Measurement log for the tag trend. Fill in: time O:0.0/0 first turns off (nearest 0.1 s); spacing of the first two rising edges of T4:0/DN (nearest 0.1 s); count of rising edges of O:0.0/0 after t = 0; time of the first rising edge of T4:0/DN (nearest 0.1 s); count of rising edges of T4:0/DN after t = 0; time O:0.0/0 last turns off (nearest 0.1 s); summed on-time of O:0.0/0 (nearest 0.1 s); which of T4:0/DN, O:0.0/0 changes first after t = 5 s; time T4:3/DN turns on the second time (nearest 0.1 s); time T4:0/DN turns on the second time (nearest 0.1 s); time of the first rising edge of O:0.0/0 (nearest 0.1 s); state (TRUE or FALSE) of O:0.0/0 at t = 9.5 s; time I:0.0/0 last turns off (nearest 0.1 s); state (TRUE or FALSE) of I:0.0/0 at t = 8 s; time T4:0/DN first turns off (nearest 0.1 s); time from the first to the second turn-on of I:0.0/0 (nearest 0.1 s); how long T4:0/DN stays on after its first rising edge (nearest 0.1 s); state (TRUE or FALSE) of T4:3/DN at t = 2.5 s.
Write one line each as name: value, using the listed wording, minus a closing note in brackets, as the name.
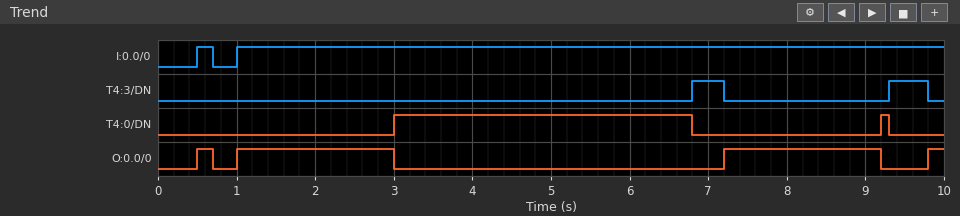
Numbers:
time O:0.0/0 first turns off: 0.7 s
spacing of the first two rising edges of T4:0/DN: 6.2 s
count of rising edges of O:0.0/0 after t = 0: 4
time of the first rising edge of T4:0/DN: 3.0 s
count of rising edges of T4:0/DN after t = 0: 2
time O:0.0/0 last turns off: 9.2 s
summed on-time of O:0.0/0: 4.4 s
which of T4:0/DN, O:0.0/0 changes first after t = 5 s: T4:0/DN
time T4:3/DN turns on the second time: 9.3 s
time T4:0/DN turns on the second time: 9.2 s
time of the first rising edge of O:0.0/0: 0.5 s
state (TRUE or FALSE) of O:0.0/0 at t = 9.5 s: FALSE
time I:0.0/0 last turns off: 0.7 s
state (TRUE or FALSE) of I:0.0/0 at t = 8 s: TRUE
time T4:0/DN first turns off: 6.8 s
time from the first to the second turn-on of I:0.0/0: 0.5 s
how long T4:0/DN stays on after its first rising edge: 3.8 s
state (TRUE or FALSE) of T4:3/DN at t = 2.5 s: FALSE
